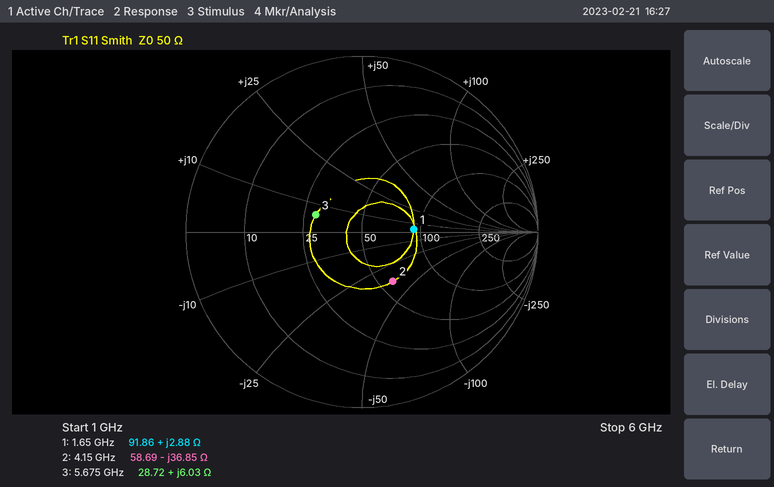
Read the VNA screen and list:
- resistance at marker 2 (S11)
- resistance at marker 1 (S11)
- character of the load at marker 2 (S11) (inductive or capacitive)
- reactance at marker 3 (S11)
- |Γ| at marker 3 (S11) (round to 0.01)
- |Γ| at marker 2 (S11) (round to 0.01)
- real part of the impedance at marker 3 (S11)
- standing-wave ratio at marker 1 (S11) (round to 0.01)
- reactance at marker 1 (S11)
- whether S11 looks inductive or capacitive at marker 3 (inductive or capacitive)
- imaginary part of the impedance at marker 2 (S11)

58.69 Ω
91.86 Ω
capacitive
+6.03 Ω
0.28
0.33
28.72 Ω
1.84
+2.88 Ω
inductive
-36.85 Ω
